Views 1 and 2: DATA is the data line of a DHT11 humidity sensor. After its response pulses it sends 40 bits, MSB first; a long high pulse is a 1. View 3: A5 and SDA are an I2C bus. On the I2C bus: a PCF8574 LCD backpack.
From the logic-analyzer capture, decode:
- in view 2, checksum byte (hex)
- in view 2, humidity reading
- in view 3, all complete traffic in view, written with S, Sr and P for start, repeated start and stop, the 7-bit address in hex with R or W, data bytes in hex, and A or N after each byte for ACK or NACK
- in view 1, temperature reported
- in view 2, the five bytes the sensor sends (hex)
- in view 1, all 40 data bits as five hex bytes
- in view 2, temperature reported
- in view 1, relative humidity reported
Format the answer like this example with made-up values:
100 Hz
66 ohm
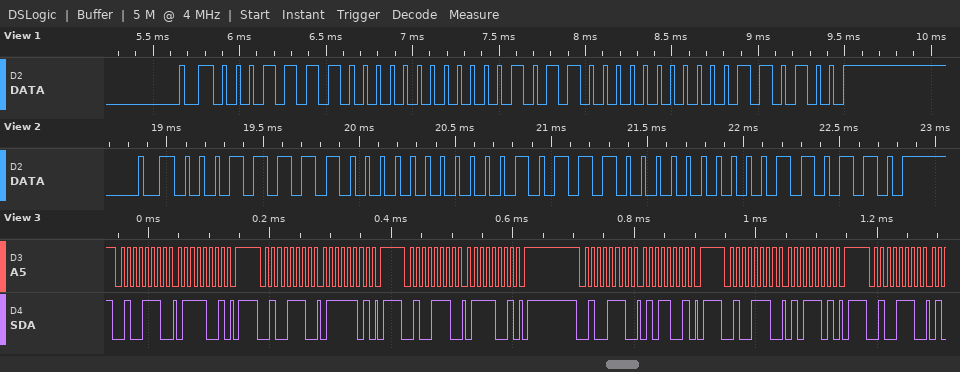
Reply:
0x36
31 %
S 27W A 79 A P S 27W A 7D A P S 27W A 79 A P S 27W A 59 A P S 27W A 5D A P S 27W A
22.0 °C
1F 00 17 00 36
1E 00 16 00 34
23.0 °C
30 %
